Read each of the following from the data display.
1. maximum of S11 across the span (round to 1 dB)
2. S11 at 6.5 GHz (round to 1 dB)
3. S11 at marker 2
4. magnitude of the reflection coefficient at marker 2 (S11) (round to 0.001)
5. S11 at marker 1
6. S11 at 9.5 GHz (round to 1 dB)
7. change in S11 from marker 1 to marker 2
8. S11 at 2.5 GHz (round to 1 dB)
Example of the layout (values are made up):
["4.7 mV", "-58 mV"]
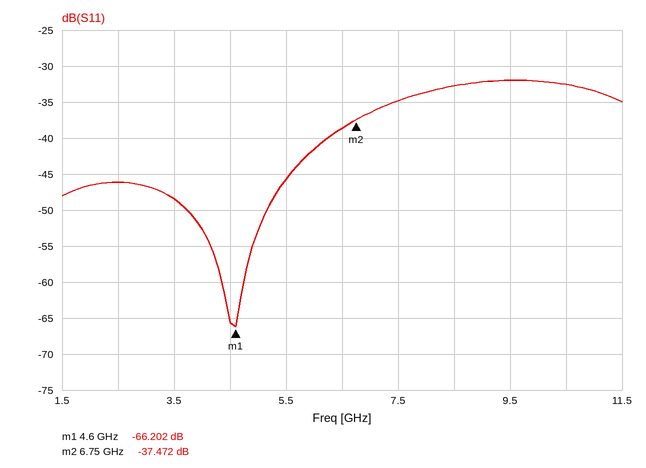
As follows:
["-32 dB", "-39 dB", "-37.472 dB", "0.013", "-66.202 dB", "-32 dB", "28.730 dB", "-46 dB"]
